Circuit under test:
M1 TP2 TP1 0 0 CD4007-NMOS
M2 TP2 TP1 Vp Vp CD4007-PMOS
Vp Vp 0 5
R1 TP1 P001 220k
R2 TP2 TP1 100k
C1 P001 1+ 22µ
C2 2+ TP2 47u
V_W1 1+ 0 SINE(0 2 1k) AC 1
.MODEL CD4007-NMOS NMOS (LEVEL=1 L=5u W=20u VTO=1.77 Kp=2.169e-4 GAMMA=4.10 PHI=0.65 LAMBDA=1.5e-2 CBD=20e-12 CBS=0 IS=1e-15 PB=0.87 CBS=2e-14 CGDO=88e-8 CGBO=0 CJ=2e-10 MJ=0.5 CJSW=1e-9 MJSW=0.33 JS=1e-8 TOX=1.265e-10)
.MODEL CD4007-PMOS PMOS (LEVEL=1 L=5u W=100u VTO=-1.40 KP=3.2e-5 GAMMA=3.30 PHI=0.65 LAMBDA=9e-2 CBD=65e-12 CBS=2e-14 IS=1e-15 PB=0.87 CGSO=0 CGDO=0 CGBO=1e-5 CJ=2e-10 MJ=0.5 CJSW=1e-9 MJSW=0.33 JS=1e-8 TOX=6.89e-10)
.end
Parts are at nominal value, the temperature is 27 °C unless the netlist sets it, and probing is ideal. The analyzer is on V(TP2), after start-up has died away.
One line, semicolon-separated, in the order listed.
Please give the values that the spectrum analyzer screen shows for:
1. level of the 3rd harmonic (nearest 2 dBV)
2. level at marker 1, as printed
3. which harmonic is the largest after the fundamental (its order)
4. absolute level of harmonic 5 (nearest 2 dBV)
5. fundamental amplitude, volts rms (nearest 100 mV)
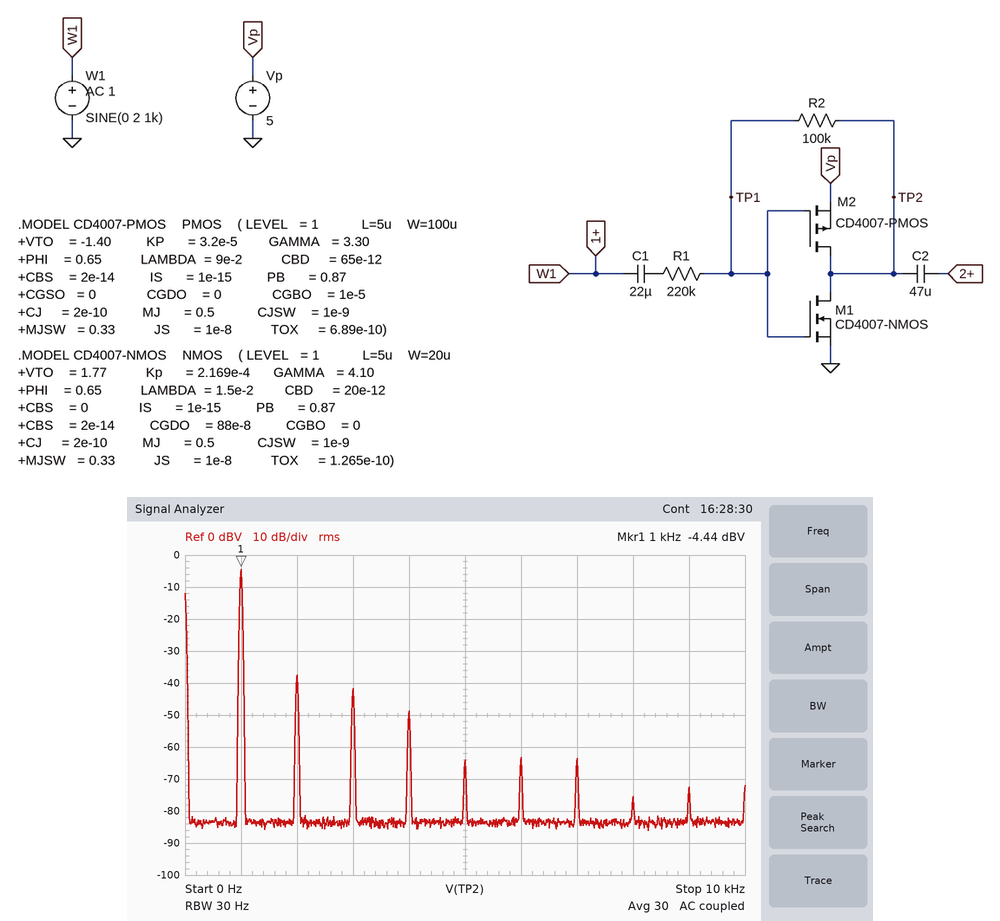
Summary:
-42 dBV; -4.44 dBV; 2; -64 dBV; 600 mV
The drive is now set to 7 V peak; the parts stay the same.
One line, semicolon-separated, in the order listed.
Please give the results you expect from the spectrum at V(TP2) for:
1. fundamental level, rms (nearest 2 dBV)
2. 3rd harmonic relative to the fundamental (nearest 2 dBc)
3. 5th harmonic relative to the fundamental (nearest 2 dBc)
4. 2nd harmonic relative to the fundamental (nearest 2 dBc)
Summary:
4 dBV; -22 dBc; -38 dBc; -14 dBc
